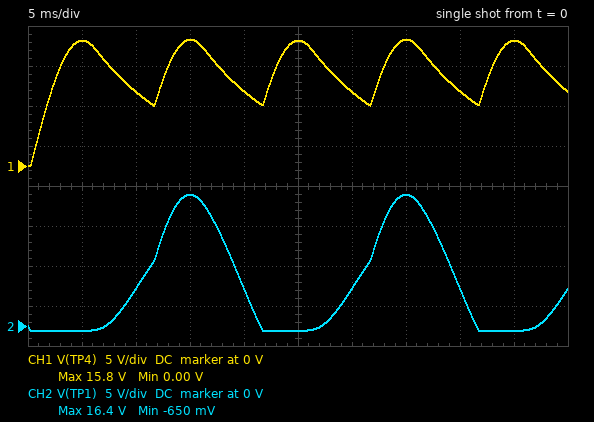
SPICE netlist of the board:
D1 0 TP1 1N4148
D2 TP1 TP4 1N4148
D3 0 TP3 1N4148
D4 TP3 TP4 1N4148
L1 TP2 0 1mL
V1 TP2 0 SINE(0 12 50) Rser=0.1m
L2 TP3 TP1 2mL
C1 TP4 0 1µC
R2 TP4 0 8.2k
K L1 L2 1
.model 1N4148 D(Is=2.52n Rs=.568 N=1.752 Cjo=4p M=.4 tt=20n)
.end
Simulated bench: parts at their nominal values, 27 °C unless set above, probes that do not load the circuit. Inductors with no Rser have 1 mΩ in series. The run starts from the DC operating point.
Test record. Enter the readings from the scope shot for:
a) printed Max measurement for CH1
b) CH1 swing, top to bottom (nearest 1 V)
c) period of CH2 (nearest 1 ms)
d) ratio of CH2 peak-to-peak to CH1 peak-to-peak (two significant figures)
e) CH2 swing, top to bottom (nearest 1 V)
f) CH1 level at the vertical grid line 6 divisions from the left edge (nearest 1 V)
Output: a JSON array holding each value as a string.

["15.8 V", "16 V", "20 ms", "1.1", "17 V", "9 V"]
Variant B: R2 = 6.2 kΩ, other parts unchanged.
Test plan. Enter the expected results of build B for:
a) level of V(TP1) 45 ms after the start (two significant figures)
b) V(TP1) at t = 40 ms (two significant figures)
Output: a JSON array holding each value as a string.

["-630 mV", "4.0 V"]
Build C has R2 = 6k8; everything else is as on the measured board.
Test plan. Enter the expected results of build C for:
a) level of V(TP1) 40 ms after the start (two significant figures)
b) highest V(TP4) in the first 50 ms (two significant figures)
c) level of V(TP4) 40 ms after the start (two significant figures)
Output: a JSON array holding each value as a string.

["4.2 V", "16 V", "8.5 V"]
